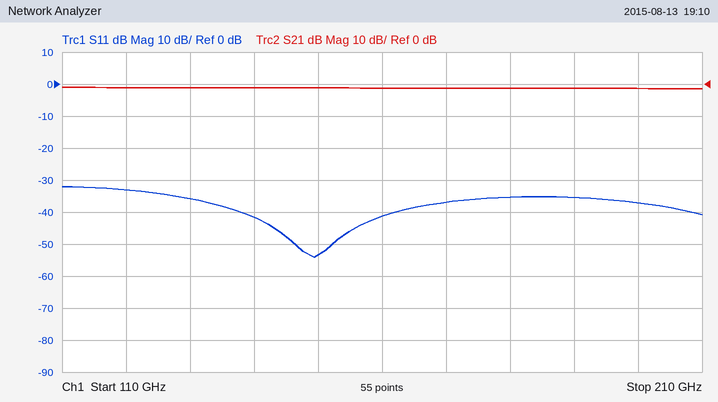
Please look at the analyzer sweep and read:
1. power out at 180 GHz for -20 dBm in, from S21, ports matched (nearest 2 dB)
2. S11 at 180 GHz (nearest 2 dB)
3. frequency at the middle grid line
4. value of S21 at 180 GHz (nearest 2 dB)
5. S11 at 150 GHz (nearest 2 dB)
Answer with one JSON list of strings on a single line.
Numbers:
["-22 dBm", "-36 dB", "160 GHz", "-2 dB", "-54 dB"]
